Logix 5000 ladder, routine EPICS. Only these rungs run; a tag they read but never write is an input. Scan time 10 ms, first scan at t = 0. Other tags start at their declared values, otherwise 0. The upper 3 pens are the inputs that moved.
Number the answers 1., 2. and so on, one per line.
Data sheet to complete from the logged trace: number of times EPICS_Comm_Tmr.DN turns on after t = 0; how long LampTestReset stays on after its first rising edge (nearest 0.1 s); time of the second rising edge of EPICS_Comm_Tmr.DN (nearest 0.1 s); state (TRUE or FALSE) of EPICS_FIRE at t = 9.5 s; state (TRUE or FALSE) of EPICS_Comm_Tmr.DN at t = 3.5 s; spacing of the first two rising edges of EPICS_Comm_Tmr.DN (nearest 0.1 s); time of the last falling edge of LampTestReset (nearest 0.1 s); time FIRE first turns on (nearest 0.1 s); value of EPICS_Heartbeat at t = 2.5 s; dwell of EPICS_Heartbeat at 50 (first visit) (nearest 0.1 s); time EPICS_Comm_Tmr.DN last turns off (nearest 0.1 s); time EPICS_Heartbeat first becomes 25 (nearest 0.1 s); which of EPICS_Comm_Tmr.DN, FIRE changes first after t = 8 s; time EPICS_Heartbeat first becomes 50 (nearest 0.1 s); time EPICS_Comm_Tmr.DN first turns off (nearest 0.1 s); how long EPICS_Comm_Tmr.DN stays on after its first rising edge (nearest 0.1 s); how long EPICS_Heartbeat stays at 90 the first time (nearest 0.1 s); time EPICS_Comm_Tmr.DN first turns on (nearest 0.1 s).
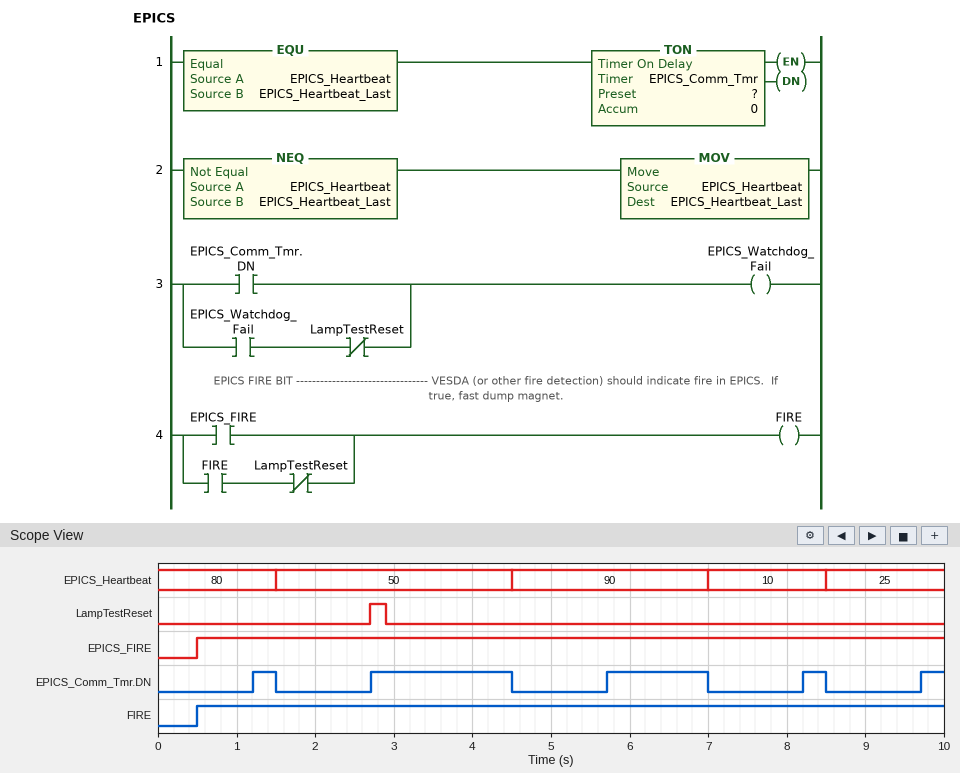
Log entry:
1. 5
2. 0.2 s
3. 2.7 s
4. TRUE
5. TRUE
6. 1.5 s
7. 2.9 s
8. 0.5 s
9. 50
10. 3.0 s
11. 8.5 s
12. 8.5 s
13. EPICS_Comm_Tmr.DN
14. 1.5 s
15. 1.5 s
16. 0.3 s
17. 2.5 s
18. 1.2 s
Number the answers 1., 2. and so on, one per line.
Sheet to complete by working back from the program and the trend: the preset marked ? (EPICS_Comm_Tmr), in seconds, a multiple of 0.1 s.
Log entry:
1. 1.2 s
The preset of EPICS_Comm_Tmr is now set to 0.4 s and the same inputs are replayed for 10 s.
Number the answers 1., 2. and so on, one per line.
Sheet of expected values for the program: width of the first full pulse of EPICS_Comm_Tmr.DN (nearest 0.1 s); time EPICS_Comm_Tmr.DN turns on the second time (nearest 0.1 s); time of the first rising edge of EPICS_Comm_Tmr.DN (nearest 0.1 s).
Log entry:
1. 1.1 s
2. 1.9 s
3. 0.4 s
